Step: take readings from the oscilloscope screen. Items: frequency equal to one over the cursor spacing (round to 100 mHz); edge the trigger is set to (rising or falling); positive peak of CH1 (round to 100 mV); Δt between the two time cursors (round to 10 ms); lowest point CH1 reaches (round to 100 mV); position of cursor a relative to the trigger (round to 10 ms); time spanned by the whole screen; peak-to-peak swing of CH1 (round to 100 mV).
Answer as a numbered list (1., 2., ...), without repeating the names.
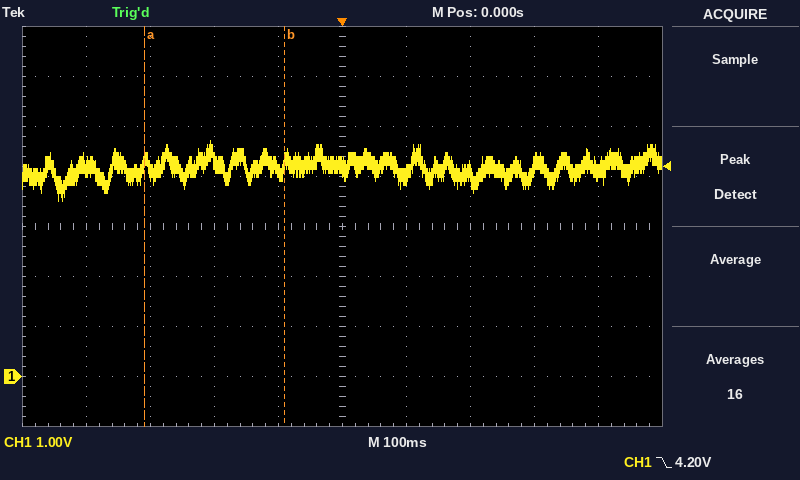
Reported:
1. 4.5 Hz
2. falling
3. 4.7 V
4. 220 ms
5. 3.5 V
6. -310 ms
7. 1 s
8. 1.2 V
